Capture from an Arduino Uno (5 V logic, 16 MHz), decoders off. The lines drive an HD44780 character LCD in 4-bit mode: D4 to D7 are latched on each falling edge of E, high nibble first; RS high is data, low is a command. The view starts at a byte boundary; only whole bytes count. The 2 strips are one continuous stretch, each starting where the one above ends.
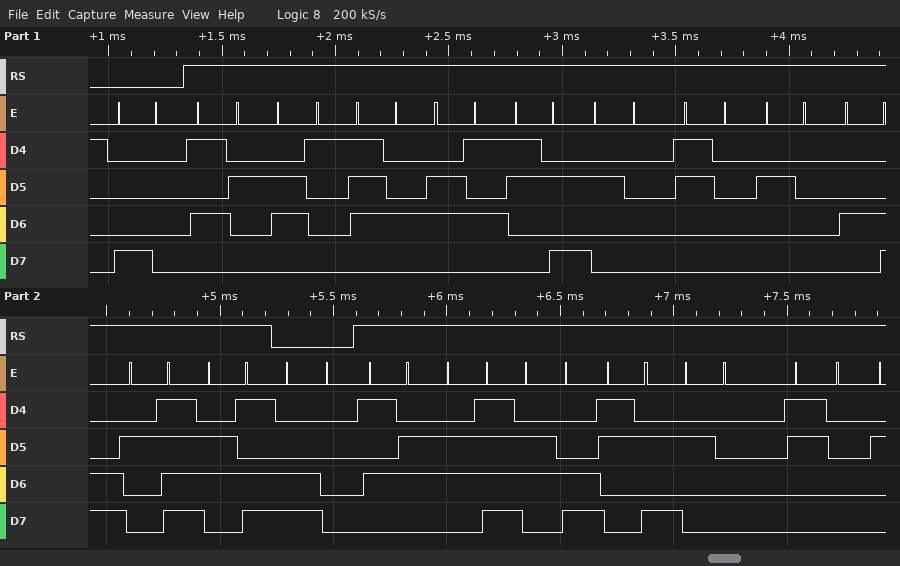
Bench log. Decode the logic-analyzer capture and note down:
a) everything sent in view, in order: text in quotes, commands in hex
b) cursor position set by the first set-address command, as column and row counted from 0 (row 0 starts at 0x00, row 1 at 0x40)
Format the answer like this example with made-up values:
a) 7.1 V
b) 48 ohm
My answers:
a) 0x80 "Rate: 0 L/m" 0xC0 "Vol: 0"
b) column 0, row 0
